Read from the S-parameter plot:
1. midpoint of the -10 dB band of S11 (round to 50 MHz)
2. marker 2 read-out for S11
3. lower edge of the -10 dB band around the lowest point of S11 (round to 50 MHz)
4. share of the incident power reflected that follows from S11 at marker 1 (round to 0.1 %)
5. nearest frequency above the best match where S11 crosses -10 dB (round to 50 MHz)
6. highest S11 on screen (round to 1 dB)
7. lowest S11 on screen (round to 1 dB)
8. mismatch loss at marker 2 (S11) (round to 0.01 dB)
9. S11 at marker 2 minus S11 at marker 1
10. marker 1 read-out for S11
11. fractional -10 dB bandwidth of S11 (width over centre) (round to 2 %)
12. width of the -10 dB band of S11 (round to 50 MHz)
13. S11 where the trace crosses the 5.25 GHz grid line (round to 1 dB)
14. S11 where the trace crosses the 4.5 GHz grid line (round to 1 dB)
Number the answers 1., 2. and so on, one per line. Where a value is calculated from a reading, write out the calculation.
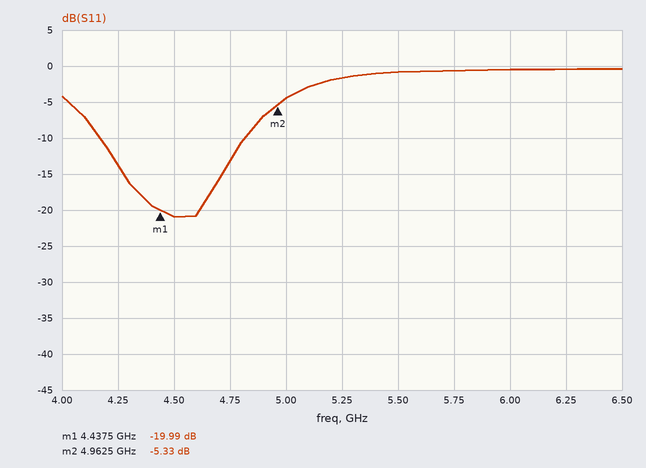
1. 4.50 GHz
2. -5.33 dB
3. 4.15 GHz
4. 10^(-19.99/10) ≈ 1.0 %
5. 4.80 GHz
6. 0 dB
7. -21 dB
8. −10 log10(1 − 10^(-5.33/10)) ≈ 1.51 dB
9. -5.33 − (-19.99) = 14.66 dB
10. -19.99 dB
11. 650 MHz / 4.475 GHz ≈ 14 %
12. 4.80 GHz − 4.15 GHz = 650 MHz
13. -2 dB
14. -21 dB
